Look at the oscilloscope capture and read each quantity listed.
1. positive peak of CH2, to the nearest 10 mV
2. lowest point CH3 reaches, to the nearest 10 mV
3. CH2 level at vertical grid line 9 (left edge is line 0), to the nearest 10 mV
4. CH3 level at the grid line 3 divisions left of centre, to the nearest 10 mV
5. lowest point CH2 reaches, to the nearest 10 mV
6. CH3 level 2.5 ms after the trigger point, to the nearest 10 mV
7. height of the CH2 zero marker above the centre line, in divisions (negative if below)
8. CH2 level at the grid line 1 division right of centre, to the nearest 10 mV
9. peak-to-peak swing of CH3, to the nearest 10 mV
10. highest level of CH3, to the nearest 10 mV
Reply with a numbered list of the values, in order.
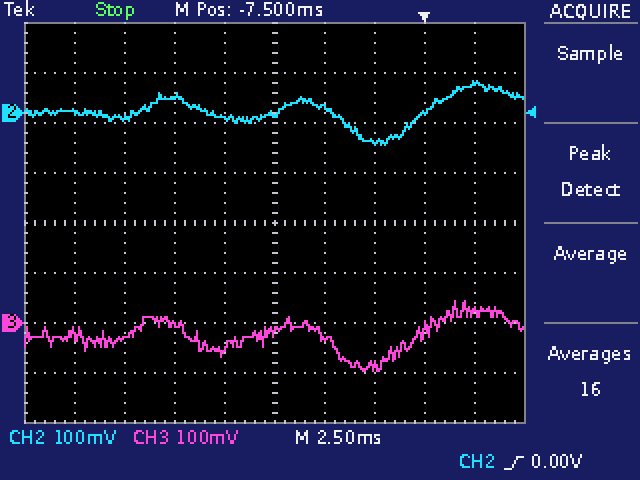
1. 60 mV
2. -100 mV
3. 60 mV
4. -30 mV
5. -60 mV
6. 20 mV
7. +2.2 div
8. 10 mV
9. 140 mV
10. 40 mV
